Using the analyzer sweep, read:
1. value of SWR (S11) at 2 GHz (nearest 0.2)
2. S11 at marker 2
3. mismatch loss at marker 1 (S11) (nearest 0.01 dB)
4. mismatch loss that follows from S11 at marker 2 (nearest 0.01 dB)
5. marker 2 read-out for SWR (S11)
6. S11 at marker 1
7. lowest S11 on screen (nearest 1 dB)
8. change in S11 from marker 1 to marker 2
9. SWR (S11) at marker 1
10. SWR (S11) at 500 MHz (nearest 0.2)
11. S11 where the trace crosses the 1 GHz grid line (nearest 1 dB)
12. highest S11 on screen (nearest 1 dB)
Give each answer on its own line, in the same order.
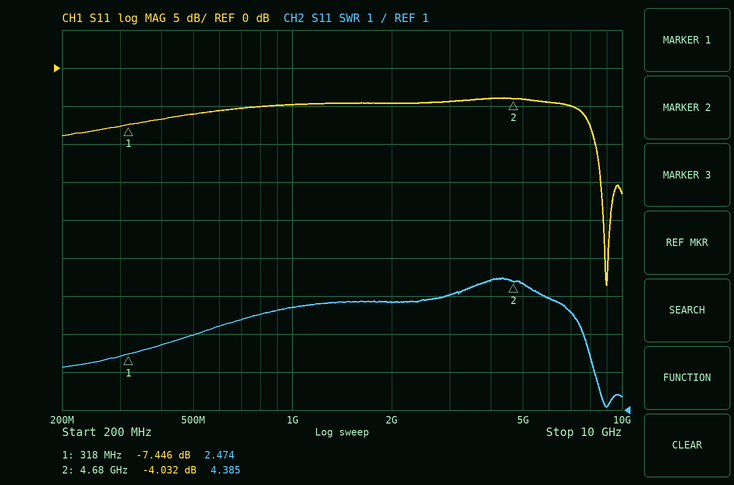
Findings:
3.8
-4.032 dB
0.86 dB
2.18 dB
4.385
-7.446 dB
-29 dB
3.414 dB
2.474
3.0
-5 dB
-4 dB
